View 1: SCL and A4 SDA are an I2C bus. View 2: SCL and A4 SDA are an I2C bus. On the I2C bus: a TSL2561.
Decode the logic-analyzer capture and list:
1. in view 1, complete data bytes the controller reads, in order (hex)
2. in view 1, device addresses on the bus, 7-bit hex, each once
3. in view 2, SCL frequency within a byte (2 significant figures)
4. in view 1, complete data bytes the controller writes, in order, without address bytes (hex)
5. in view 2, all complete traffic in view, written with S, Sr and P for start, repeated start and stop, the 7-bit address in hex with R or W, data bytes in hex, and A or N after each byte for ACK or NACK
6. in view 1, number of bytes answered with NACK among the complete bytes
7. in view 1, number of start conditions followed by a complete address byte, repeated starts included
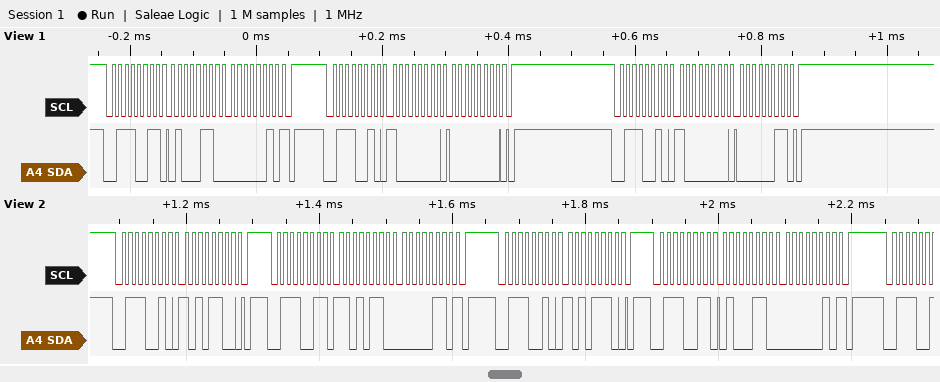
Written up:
46 02
0x39
100 kHz
80 00 80 03
S 39W A AC A P S 39R A D6 A 06 N P S 39W A AE A P S 39R A 46 A 02 N P
1
3
